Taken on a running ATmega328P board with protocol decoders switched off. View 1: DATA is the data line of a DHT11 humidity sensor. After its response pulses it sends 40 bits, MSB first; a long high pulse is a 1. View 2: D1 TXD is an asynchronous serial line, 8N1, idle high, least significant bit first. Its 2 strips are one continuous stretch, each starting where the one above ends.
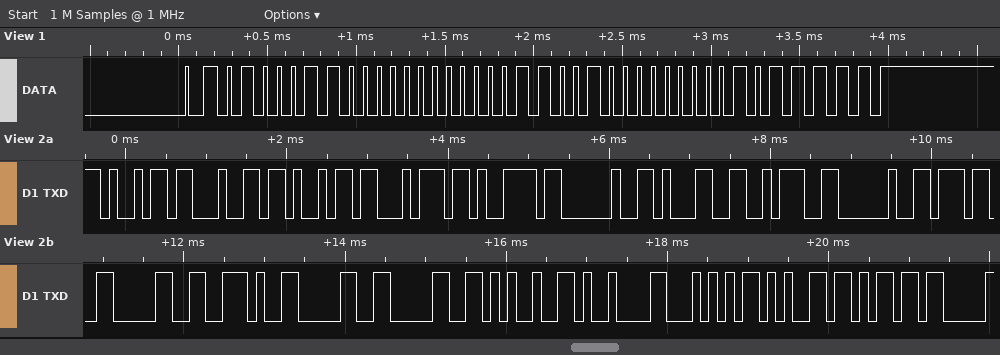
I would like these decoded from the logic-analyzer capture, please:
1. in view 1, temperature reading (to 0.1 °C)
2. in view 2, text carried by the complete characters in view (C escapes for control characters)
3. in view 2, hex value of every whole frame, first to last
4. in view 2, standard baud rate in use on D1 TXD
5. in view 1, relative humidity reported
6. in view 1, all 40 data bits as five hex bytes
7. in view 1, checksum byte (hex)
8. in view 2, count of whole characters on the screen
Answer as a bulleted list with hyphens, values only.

- 25.0 °C
- "idity 1: 70.00%\tTem"
- 0x69 0x64 0x69 0x74 0x79 0x20 0x31 0x3A 0x20 0x37 0x30 0x2E 0x30 0x30 0x25 0x09 0x54 0x65 0x6D
- 9600 baud
- 70 %
- 46 00 19 00 5F
- 0x5F
- 19
